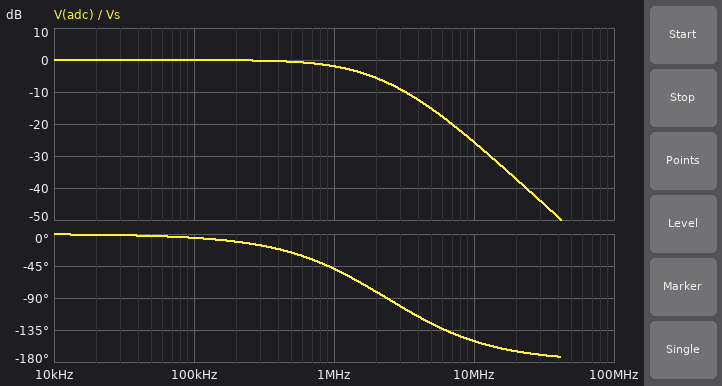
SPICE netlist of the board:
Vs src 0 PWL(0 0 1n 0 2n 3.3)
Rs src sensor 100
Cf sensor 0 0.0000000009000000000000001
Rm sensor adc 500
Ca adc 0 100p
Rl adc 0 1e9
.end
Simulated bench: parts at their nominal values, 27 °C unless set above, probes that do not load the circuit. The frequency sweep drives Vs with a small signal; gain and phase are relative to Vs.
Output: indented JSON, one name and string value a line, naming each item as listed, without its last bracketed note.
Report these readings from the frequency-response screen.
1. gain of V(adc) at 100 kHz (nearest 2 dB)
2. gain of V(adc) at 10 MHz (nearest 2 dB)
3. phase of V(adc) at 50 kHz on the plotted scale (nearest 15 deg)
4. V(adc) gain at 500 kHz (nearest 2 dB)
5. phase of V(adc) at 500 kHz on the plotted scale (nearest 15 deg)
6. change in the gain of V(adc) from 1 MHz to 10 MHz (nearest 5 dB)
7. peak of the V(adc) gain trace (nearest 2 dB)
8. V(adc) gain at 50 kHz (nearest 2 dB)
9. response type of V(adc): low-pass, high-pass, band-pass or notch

{
  "gain of V(adc) at 100 kHz": "0 dB",
  "gain of V(adc) at 10 MHz": "-26 dB",
  "phase of V(adc) at 50 kHz on the plotted scale": "0 deg",
  "V(adc) gain at 500 kHz": "0 dB",
  "phase of V(adc) at 500 kHz on the plotted scale": "-30 deg",
  "change in the gain of V(adc) from 1 MHz to 10 MHz": "-25 dB",
  "peak of the V(adc) gain trace": "0 dB",
  "V(adc) gain at 50 kHz": "0 dB",
  "response type of V(adc): low-pass, high-pass, band-pass or notch": "low-pass"
}
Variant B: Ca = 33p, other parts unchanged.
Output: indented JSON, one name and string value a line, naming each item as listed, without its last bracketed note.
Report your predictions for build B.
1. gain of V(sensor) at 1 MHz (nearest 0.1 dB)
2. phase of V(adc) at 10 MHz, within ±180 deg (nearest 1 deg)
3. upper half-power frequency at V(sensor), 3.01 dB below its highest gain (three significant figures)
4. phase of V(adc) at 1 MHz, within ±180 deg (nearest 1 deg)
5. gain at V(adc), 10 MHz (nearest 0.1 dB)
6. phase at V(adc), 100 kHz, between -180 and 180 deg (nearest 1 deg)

{
  "gain of V(sensor) at 1 MHz": "-1.3 dB",
  "phase of V(adc) at 10 MHz, within ±180 deg": "-125 deg",
  "upper half-power frequency at V(sensor), 3.01 dB below its highest gain": "1.70 MHz",
  "phase of V(adc) at 1 MHz, within ±180 deg": "-36 deg",
  "gain at V(adc), 10 MHz": "-18.5 dB",
  "phase at V(adc), 100 kHz, between -180 and 180 deg": "-4 deg"
}
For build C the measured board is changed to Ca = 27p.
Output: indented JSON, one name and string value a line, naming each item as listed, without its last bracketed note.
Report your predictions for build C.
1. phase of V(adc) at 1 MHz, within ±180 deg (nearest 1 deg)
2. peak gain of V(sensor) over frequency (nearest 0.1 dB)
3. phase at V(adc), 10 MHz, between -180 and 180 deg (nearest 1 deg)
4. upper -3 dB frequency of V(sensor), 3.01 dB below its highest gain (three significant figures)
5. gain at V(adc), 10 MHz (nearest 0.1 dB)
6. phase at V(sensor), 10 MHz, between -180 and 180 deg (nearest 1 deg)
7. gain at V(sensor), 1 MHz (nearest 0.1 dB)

{
  "phase of V(adc) at 1 MHz, within ±180 deg": "-35 deg",
  "peak gain of V(sensor) over frequency": "0 dB",
  "phase at V(adc), 10 MHz, between -180 and 180 deg": "-120 deg",
  "upper -3 dB frequency of V(sensor), 3.01 dB below its highest gain": "1.71 MHz",
  "gain at V(adc), 10 MHz": "-17.7 dB",
  "phase at V(sensor), 10 MHz, between -180 and 180 deg": "-79 deg",
  "gain at V(sensor), 1 MHz": "-1.3 dB"
}
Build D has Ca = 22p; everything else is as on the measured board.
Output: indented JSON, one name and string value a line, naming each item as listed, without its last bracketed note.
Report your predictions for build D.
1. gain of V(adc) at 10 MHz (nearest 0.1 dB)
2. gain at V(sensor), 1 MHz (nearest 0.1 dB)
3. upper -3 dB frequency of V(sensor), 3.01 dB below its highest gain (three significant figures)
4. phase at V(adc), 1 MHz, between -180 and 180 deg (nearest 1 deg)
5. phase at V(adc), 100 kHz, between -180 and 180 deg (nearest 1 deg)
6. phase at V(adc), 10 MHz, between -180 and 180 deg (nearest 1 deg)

{
  "gain of V(adc) at 10 MHz": "-17.0 dB",
  "gain at V(sensor), 1 MHz": "-1.3 dB",
  "upper -3 dB frequency of V(sensor), 3.01 dB below its highest gain": "1.72 MHz",
  "phase at V(adc), 1 MHz, between -180 and 180 deg": "-34 deg",
  "phase at V(adc), 100 kHz, between -180 and 180 deg": "-4 deg",
  "phase at V(adc), 10 MHz, between -180 and 180 deg": "-114 deg"
}
